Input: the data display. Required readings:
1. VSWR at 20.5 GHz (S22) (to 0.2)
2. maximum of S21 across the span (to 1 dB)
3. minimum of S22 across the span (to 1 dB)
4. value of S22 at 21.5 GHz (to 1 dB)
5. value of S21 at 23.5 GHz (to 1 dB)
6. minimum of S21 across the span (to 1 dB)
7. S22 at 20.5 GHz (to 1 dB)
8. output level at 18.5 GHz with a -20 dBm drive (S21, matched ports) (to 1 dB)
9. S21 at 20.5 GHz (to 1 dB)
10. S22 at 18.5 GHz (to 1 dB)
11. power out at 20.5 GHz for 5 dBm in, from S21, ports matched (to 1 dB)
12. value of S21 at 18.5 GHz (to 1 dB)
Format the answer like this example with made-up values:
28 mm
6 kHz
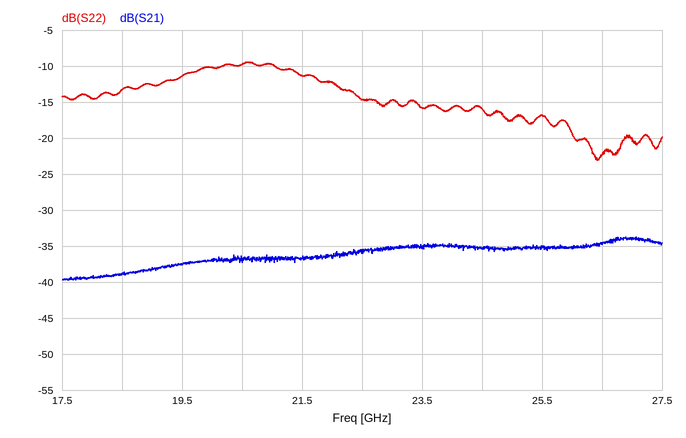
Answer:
2.0
-34 dB
-23 dB
-11 dB
-35 dB
-40 dB
-10 dB
-59 dBm
-37 dB
-13 dB
-32 dBm
-39 dB
